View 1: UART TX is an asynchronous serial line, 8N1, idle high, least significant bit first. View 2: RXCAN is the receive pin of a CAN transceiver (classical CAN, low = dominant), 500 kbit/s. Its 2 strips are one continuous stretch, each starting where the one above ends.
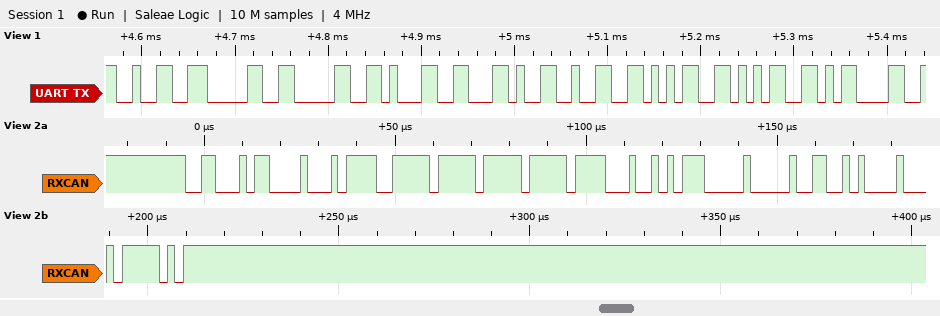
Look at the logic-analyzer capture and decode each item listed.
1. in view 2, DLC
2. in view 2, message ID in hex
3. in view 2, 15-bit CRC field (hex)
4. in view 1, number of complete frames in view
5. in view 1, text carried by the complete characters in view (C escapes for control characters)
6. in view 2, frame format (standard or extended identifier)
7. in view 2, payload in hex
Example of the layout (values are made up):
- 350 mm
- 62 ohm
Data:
- 8
- 0x316
- 0x045F
- 9
- "2001,255\r"
- standard
- BC FF FF FF 12 B8 00 65
